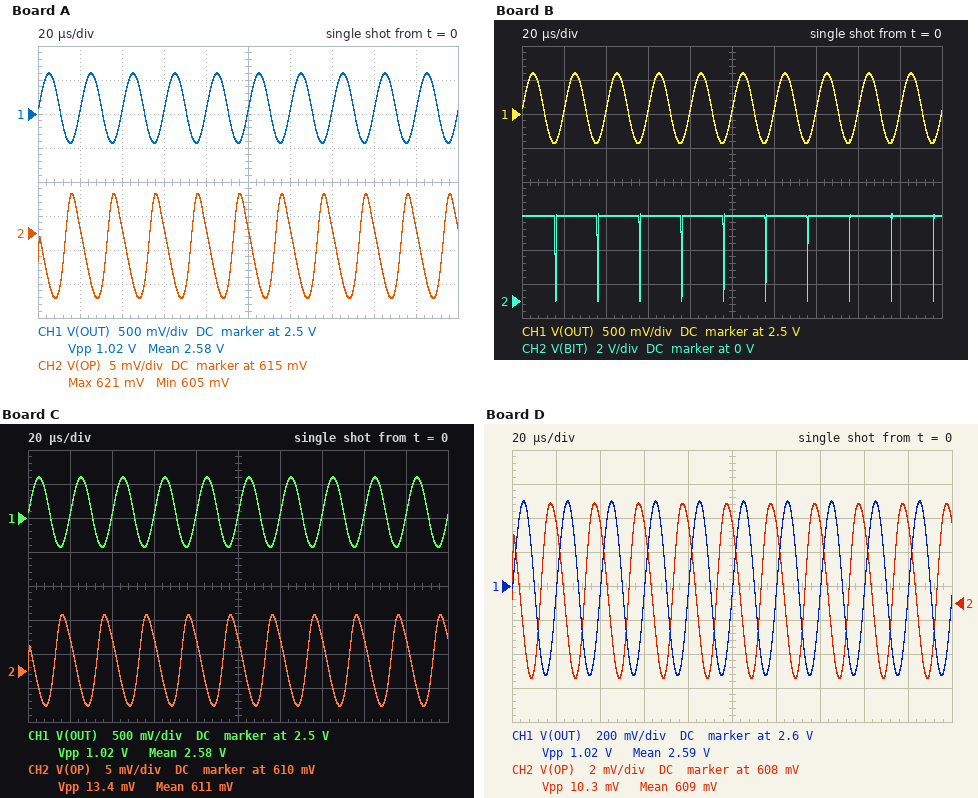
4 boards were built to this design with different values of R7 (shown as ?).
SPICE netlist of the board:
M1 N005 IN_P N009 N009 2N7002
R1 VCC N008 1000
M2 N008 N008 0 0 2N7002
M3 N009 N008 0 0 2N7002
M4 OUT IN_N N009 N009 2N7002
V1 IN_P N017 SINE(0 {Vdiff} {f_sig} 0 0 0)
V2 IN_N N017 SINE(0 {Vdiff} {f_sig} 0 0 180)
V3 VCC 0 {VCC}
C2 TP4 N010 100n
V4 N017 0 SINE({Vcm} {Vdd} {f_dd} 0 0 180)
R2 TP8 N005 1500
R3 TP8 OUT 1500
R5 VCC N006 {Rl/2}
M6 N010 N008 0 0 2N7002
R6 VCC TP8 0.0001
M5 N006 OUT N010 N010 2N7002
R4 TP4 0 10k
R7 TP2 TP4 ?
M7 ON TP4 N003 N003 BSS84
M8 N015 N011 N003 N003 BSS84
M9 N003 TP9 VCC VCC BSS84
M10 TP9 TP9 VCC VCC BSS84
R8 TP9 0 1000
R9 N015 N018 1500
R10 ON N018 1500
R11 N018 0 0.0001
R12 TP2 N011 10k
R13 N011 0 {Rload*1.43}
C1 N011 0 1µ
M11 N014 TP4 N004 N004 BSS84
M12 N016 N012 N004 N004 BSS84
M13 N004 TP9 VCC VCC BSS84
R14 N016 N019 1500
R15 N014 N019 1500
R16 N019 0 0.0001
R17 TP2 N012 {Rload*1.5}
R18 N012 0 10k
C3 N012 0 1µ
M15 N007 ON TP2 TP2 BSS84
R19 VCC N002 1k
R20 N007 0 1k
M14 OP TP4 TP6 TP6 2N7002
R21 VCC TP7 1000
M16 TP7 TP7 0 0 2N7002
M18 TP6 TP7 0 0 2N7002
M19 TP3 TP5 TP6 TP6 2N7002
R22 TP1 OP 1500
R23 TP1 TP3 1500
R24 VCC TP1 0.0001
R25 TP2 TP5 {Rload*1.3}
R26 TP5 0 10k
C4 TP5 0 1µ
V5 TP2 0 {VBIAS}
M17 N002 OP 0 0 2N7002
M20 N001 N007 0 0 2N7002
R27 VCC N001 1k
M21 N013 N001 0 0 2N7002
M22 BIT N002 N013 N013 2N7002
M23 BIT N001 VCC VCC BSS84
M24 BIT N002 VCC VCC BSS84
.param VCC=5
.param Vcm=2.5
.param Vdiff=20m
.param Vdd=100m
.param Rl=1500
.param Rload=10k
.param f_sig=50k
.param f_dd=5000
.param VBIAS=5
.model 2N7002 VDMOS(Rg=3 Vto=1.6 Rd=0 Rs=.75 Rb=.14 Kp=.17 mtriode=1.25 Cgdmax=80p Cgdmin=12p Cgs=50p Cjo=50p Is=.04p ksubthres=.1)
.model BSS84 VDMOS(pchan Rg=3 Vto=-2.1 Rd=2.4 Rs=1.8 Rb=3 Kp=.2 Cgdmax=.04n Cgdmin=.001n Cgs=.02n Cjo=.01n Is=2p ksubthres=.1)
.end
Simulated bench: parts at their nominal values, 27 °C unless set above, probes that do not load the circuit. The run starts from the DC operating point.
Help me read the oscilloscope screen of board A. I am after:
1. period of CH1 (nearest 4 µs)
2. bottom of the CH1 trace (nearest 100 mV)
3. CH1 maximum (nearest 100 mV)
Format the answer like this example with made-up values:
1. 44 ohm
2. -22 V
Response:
1. 20 µs
2. 2.1 V
3. 3.1 V
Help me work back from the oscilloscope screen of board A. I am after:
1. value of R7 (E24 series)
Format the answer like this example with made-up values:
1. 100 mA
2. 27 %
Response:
1. 5.1 kΩ
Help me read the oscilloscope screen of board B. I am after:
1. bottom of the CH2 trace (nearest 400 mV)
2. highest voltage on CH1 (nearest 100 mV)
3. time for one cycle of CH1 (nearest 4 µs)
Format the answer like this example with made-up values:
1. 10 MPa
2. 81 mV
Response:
1. 0 V
2. 3.1 V
3. 20 µs
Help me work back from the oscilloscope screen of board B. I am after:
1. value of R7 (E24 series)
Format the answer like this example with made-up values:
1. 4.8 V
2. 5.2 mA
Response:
1. 5.6 kΩ
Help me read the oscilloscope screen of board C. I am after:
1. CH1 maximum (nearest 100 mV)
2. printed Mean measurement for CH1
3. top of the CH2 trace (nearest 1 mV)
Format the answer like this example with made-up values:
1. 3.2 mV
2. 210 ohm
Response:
1. 3.1 V
2. 2.58 V
3. 618 mV
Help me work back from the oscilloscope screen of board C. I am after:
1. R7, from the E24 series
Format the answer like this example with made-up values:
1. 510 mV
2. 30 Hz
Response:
1. 4.7 kΩ
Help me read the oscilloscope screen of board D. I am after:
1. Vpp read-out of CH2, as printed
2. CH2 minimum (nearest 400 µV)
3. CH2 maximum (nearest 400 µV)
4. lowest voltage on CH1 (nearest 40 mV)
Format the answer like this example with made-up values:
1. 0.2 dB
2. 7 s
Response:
1. 10.3 mV
2. 603.6 mV
3. 614.0 mV
4. 2.08 V
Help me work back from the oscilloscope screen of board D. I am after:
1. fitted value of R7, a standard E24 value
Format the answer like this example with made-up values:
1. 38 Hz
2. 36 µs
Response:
1. 3.6 kΩ
